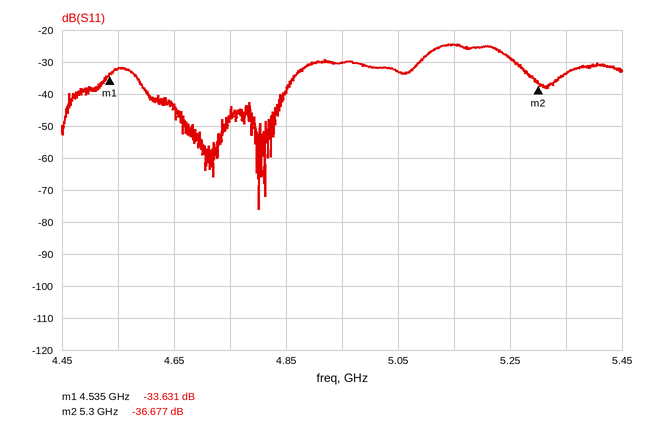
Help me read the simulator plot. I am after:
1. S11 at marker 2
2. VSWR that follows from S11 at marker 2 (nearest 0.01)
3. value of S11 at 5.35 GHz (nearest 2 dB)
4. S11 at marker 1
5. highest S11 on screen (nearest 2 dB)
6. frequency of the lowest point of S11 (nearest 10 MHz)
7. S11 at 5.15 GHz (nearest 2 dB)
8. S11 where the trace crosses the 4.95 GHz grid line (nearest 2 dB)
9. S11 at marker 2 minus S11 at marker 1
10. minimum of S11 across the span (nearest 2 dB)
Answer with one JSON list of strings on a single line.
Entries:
["-36.677 dB", "1.03", "-34 dB", "-33.631 dB", "-24 dB", "4.80 GHz", "-24 dB", "-30 dB", "-3.046 dB", "-76 dB"]
